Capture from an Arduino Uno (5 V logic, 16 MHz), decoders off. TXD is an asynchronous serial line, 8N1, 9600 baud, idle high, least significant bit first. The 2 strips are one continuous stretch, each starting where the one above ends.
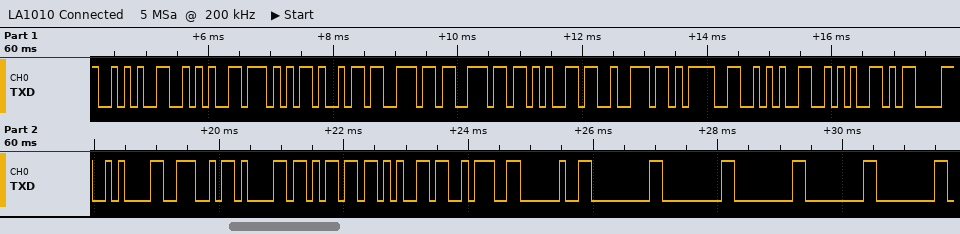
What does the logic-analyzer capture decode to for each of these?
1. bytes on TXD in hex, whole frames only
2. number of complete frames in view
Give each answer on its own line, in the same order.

0x2A 0x2A 0x57 0x69 0x6E 0x6E 0x65 0x72 0x3D 0x2A 0x2A 0x0D 0x0A 0x4E 0x61 0x6D 0x65 0x3A 0x20 0x00 0x00 0x00 0x00 0x00
24
